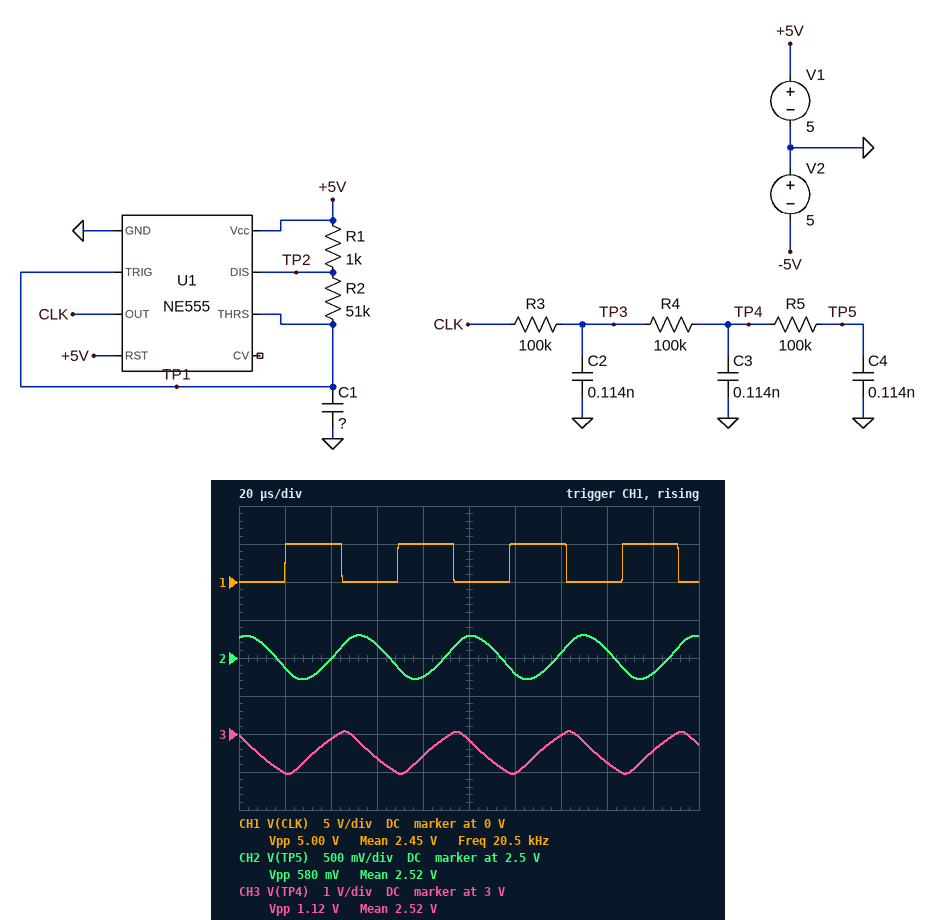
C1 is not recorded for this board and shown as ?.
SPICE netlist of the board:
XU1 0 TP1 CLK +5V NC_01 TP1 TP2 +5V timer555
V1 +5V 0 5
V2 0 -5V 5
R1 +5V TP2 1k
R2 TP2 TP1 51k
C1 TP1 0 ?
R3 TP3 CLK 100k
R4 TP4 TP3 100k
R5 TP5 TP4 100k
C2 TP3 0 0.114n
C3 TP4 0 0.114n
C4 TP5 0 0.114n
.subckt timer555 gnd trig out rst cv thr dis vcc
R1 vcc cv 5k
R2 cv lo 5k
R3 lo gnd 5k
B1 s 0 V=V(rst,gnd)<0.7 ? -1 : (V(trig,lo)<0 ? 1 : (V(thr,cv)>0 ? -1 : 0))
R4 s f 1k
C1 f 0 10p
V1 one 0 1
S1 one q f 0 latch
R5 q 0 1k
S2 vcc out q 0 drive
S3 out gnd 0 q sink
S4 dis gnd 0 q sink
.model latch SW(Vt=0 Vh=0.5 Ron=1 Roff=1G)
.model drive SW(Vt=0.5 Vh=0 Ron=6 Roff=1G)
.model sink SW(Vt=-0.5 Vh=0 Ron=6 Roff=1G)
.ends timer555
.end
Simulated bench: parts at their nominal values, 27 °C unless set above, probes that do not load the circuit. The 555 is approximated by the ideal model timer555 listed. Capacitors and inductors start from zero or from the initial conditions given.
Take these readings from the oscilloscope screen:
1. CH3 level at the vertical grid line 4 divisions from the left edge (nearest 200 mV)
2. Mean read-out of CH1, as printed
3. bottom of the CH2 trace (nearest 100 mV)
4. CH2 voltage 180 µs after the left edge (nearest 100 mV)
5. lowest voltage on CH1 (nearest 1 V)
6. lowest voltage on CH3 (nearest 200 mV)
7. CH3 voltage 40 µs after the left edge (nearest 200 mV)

2.4 V
2.45 V
2.2 V
2.3 V
0 V
2.0 V
2.8 V
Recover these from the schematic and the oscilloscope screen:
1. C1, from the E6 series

680 pF
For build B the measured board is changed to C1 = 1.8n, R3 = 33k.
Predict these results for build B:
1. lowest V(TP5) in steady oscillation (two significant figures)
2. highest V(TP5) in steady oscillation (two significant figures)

910 mV
4.1 V
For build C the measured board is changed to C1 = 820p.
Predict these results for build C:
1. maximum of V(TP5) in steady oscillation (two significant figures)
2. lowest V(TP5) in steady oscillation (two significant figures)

2.9 V
2.1 V
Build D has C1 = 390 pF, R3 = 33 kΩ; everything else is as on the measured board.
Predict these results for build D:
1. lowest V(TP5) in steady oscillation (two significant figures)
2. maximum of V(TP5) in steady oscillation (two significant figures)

2.3 V
2.7 V
